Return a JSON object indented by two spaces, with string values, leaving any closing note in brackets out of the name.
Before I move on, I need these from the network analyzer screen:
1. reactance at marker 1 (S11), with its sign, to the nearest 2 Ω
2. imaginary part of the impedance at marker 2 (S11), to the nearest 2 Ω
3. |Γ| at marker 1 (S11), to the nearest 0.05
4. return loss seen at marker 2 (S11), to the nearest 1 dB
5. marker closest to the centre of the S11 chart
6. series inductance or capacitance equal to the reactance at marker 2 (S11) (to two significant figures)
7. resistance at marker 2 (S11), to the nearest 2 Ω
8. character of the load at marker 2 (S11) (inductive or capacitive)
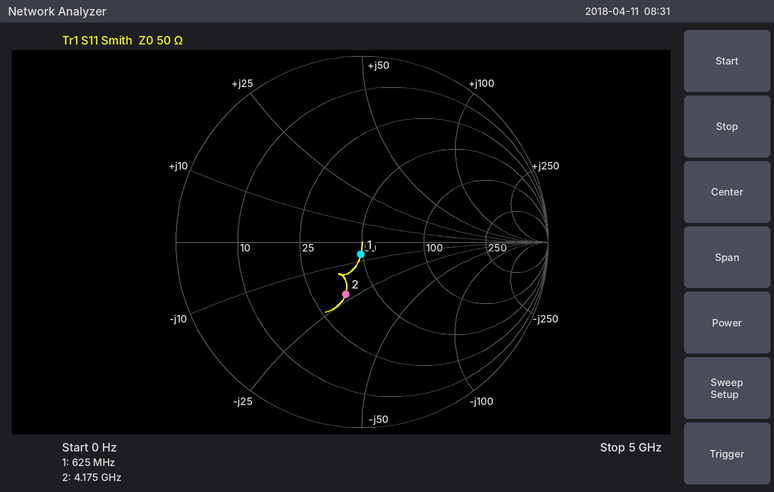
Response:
{
  "reactance at marker 1 (S11), with its sign, to the nearest 2 Ω": "-6 Ω",
  "imaginary part of the impedance at marker 2 (S11), to the nearest 2 Ω": "-22 Ω",
  "|Γ| at marker 1 (S11), to the nearest 0.05": "0.05",
  "return loss seen at marker 2 (S11), to the nearest 1 dB": "11 dB",
  "marker closest to the centre of the S11 chart": "marker 1",
  "series inductance or capacitance equal to the reactance at marker 2 (S11)": "1.7 pF",
  "resistance at marker 2 (S11), to the nearest 2 Ω": "36 Ω",
  "character of the load at marker 2 (S11)": "capacitive"
}
